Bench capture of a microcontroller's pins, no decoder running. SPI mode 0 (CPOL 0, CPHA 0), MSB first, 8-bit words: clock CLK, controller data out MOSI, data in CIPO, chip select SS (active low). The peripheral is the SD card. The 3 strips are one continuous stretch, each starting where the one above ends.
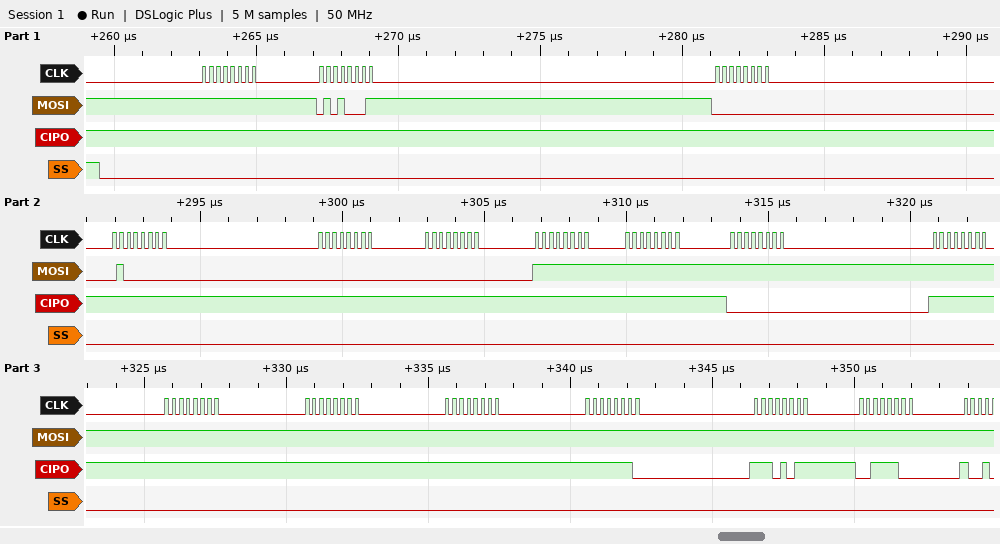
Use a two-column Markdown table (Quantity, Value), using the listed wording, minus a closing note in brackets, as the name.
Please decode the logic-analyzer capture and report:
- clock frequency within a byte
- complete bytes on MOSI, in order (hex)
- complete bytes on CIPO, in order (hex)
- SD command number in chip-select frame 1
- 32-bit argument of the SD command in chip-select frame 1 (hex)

| Quantity | Value |
|---|---|
| clock frequency within a byte | 4 MHz |
| complete bytes on MOSI, in order | FF 51 00 40 00 00 FF FF FF FF FF FF FF FF FF FF |
| complete bytes on CIPO, in order | FF FF FF FF FF FF FF FF 00 FF FF FF FF FE EB 3C |
| SD command number in chip-select frame 1 | CMD17 |
| 32-bit argument of the SD command in chip-select frame 1 | 0x00400000 |
